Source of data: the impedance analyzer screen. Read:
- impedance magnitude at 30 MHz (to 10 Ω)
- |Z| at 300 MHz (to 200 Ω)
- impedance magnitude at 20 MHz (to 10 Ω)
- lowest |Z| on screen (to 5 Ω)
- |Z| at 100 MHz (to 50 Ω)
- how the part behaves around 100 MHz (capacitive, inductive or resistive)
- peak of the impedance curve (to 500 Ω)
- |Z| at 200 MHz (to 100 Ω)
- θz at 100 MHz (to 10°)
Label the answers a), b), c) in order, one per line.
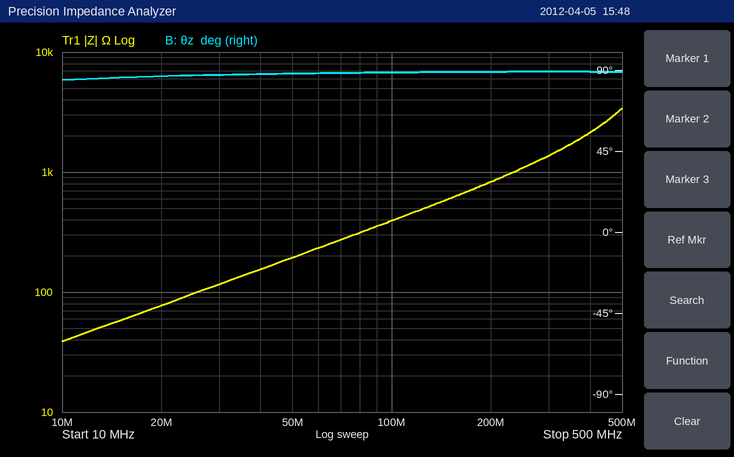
a) 120 Ω
b) 1.4 kΩ
c) 80 Ω
d) 40 Ω
e) 400 Ω
f) inductive
g) 3.5 kΩ
h) 800 Ω
i) 90°
